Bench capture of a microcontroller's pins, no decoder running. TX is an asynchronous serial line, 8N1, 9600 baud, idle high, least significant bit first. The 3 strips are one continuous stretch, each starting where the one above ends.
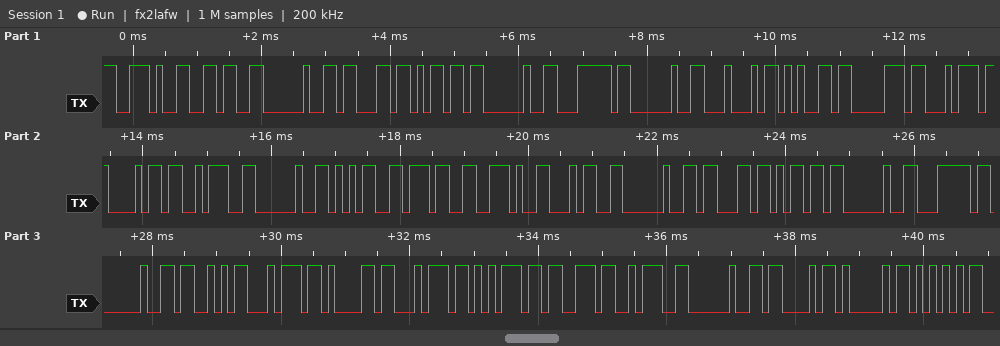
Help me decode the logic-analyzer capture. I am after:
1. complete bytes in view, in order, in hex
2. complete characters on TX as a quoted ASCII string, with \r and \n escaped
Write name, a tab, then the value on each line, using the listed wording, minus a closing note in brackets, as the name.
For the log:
complete bytes in view, in order, in hex	2E 36 20 63 6D 20 7C 20 44 65 70 74 68 3A 20 35 37 2E 34 20 63 6D 20 7C 20 53 74 61 74 75 73 3A 20 43 41 55
complete characters on TX as a quoted ASCII string, with \r and \n escaped	".6 cm | Depth: 57.4 cm | Status: CAU"
